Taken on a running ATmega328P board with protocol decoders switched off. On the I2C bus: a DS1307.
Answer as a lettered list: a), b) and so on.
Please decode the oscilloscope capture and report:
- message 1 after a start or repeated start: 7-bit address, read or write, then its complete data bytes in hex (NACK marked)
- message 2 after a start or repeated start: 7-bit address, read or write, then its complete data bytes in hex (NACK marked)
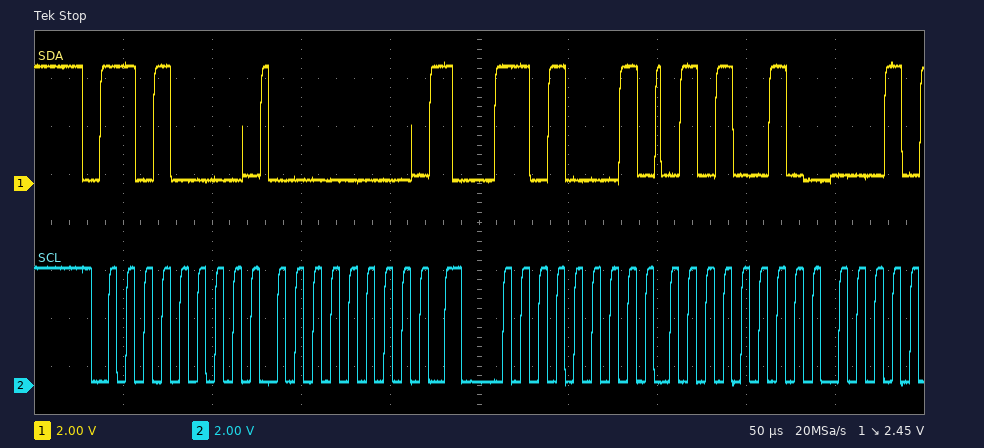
a) 0x68 write: 00
b) 0x68 read: 52
